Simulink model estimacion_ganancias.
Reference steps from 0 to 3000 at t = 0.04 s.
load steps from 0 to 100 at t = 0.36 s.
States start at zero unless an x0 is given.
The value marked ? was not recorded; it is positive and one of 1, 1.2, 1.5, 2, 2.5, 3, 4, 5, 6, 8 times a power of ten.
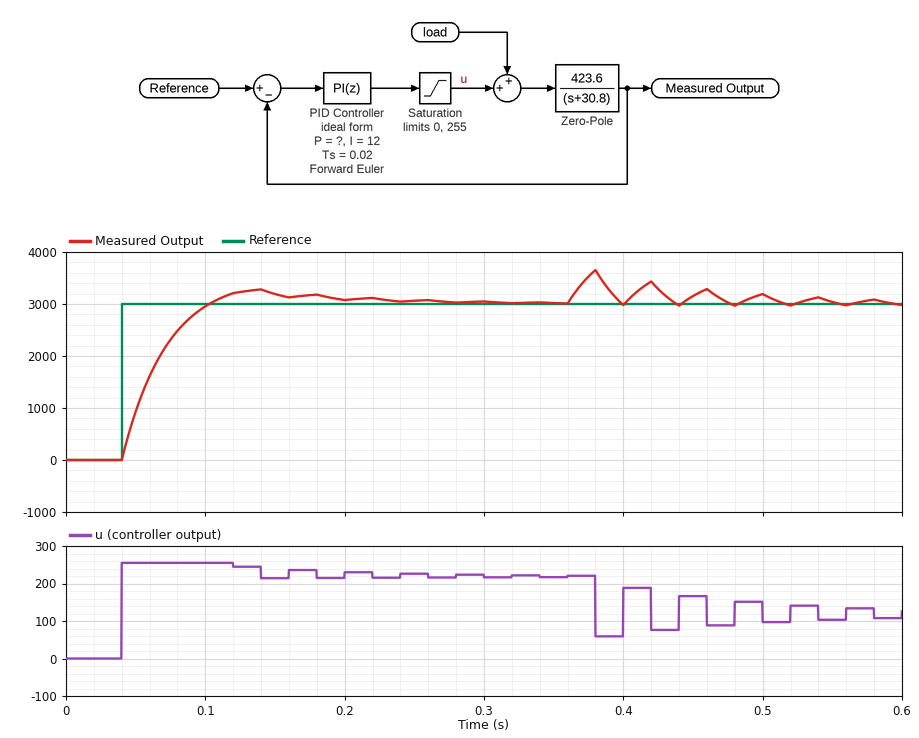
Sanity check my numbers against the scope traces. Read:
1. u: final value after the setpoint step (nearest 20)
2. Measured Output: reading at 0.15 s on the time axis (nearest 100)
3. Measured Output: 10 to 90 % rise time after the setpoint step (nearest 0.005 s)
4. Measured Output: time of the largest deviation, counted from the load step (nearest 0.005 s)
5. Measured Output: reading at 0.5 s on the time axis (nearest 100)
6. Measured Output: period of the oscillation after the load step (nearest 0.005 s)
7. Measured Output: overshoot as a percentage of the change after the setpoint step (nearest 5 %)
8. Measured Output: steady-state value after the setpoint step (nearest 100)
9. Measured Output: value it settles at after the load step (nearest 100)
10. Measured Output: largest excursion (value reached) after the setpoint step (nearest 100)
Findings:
220
3200
0.045 s
0.020 s
3200
0.040 s
10 %
3000
3000
3300
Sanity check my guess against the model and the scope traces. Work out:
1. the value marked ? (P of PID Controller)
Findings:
0.25
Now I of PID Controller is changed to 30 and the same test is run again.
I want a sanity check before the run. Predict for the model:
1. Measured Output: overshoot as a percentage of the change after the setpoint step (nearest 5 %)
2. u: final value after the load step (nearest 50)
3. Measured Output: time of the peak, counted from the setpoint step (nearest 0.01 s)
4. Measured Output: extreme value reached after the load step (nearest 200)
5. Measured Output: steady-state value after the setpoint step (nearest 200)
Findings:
15 %
100
0.22 s
3600
3000
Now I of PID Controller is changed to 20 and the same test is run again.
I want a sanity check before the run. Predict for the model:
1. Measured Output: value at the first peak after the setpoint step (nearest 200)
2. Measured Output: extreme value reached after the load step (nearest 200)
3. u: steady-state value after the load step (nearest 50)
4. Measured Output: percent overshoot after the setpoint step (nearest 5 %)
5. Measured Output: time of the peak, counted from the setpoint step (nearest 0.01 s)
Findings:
3400
3600
100
15 %
0.16 s
